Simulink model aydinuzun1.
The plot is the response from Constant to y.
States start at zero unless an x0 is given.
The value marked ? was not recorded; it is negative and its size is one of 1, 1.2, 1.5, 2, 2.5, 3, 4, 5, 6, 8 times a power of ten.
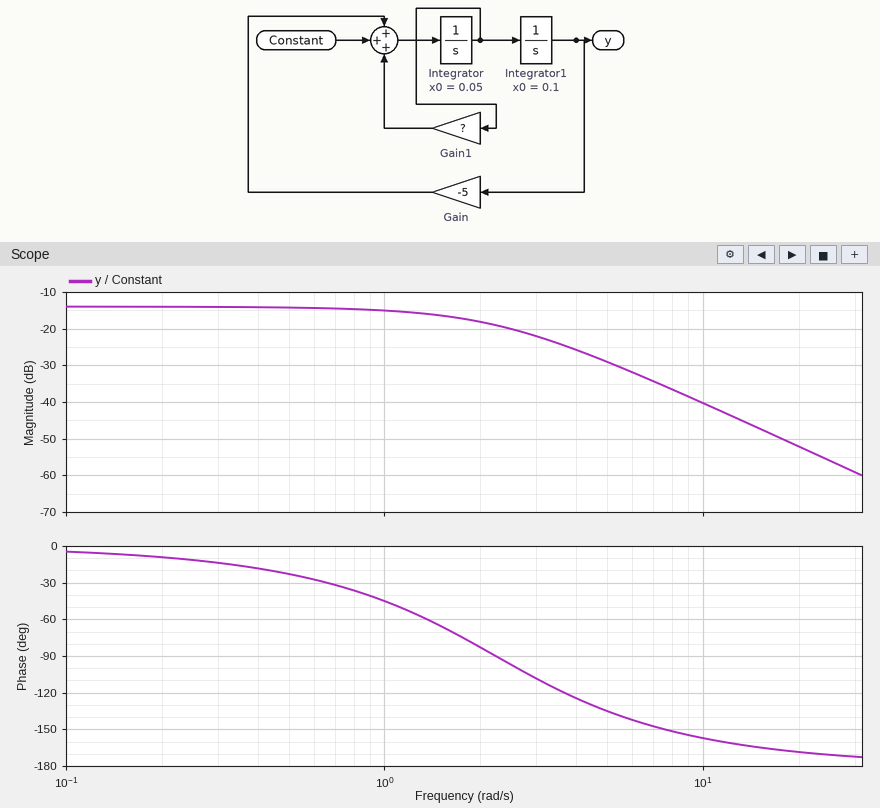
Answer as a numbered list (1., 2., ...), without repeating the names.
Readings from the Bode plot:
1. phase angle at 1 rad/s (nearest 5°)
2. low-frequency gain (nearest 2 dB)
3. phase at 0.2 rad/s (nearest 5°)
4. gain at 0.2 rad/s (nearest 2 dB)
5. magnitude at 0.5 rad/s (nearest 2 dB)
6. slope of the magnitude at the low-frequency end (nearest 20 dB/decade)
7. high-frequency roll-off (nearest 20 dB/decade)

1. -45°
2. -14 dB
3. -10°
4. -14 dB
5. -14 dB
6. 0 dB/decade
7. -40 dB/decade
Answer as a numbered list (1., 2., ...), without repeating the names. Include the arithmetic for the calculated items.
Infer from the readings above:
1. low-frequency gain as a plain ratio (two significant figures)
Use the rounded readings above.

1. 10^(-14 / 20) = 0.20
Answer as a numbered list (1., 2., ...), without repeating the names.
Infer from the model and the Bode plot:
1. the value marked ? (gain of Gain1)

1. -4
